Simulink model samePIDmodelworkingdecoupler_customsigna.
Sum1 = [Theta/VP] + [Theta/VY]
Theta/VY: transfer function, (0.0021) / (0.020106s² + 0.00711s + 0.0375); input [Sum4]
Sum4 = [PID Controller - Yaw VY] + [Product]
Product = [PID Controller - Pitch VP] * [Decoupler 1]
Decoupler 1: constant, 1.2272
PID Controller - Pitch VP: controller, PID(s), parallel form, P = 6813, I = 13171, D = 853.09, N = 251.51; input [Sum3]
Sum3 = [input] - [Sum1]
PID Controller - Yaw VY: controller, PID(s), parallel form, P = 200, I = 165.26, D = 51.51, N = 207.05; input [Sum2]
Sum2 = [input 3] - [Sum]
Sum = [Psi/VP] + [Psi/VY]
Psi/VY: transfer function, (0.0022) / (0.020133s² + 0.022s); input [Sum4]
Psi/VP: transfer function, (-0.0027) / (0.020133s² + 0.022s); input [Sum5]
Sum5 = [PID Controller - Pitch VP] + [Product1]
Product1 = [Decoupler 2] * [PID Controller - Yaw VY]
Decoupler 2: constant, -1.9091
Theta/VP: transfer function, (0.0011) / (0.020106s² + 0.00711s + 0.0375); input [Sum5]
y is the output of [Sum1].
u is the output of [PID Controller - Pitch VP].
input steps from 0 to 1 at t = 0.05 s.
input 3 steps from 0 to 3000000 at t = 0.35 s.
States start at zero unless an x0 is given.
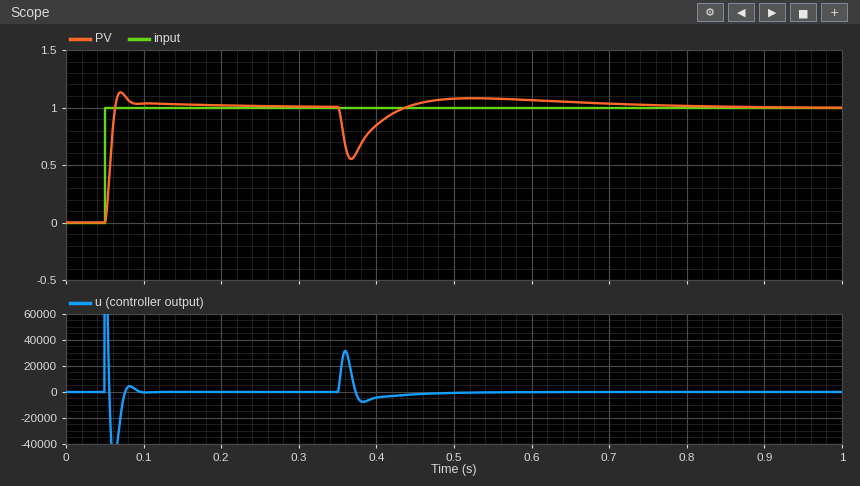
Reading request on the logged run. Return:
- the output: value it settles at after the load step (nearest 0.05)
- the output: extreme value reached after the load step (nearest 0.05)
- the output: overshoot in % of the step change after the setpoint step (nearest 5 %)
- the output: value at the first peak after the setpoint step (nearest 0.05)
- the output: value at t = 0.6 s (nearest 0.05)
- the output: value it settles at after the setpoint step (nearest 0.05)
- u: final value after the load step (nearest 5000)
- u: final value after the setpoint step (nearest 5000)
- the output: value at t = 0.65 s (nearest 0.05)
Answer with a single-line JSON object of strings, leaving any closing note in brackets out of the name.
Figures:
{"the output: value it settles at after the load step": "1.00", "the output: extreme value reached after the load step": "0.55", "the output: overshoot in % of the step change after the setpoint step": "15 %", "the output: value at the first peak after the setpoint step": "1.15", "the output: value at t = 0.6 s": "1.05", "the output: value it settles at after the setpoint step": "1.00", "u: final value after the load step": "0", "u: final value after the setpoint step": "0", "the output: value at t = 0.65 s": "1.05"}
